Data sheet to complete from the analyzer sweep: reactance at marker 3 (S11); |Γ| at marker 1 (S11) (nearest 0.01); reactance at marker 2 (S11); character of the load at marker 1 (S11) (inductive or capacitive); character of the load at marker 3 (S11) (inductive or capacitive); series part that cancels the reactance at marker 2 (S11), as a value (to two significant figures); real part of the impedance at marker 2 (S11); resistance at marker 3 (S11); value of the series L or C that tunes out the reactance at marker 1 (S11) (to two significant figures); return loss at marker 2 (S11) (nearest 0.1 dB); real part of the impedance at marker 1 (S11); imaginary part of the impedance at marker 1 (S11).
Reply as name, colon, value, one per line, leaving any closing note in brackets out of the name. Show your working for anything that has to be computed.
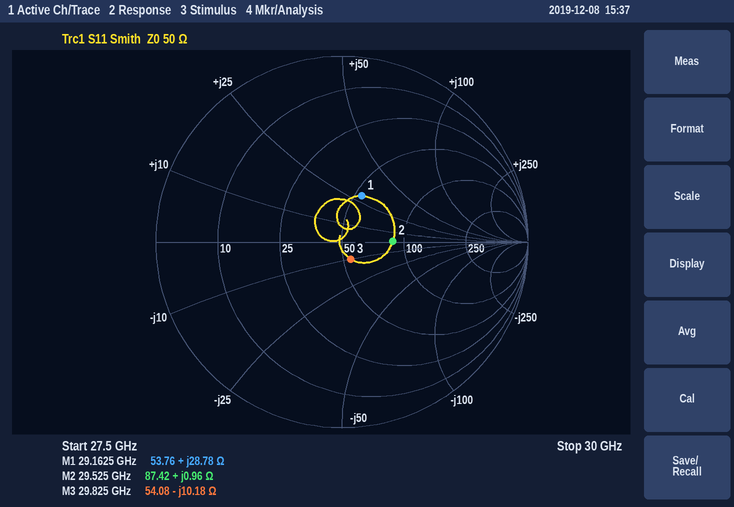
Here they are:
reactance at marker 3: -10.18 Ω
|Γ| at marker 1 (S11): 0.27
reactance at marker 2: +0.96 Ω
character of the load at marker 1 (S11): inductive
character of the load at marker 3 (S11): capacitive
series part that cancels the reactance at marker 2 (S11), as a value: C = 1/(2π × 29.525 GHz × 0.96 Ω) ≈ 5.6 pF
real part of the impedance at marker 2: 87.42 Ω
resistance at marker 3: 54.08 Ω
value of the series L or C that tunes out the reactance at marker 1 (S11): C = 1/(2π × 29.1625 GHz × 28.78 Ω) ≈ 190 fF
return loss at marker 2 (S11): 11.3 dB
real part of the impedance at marker 1: 53.76 Ω
imaginary part of the impedance at marker 1: +28.78 Ω
